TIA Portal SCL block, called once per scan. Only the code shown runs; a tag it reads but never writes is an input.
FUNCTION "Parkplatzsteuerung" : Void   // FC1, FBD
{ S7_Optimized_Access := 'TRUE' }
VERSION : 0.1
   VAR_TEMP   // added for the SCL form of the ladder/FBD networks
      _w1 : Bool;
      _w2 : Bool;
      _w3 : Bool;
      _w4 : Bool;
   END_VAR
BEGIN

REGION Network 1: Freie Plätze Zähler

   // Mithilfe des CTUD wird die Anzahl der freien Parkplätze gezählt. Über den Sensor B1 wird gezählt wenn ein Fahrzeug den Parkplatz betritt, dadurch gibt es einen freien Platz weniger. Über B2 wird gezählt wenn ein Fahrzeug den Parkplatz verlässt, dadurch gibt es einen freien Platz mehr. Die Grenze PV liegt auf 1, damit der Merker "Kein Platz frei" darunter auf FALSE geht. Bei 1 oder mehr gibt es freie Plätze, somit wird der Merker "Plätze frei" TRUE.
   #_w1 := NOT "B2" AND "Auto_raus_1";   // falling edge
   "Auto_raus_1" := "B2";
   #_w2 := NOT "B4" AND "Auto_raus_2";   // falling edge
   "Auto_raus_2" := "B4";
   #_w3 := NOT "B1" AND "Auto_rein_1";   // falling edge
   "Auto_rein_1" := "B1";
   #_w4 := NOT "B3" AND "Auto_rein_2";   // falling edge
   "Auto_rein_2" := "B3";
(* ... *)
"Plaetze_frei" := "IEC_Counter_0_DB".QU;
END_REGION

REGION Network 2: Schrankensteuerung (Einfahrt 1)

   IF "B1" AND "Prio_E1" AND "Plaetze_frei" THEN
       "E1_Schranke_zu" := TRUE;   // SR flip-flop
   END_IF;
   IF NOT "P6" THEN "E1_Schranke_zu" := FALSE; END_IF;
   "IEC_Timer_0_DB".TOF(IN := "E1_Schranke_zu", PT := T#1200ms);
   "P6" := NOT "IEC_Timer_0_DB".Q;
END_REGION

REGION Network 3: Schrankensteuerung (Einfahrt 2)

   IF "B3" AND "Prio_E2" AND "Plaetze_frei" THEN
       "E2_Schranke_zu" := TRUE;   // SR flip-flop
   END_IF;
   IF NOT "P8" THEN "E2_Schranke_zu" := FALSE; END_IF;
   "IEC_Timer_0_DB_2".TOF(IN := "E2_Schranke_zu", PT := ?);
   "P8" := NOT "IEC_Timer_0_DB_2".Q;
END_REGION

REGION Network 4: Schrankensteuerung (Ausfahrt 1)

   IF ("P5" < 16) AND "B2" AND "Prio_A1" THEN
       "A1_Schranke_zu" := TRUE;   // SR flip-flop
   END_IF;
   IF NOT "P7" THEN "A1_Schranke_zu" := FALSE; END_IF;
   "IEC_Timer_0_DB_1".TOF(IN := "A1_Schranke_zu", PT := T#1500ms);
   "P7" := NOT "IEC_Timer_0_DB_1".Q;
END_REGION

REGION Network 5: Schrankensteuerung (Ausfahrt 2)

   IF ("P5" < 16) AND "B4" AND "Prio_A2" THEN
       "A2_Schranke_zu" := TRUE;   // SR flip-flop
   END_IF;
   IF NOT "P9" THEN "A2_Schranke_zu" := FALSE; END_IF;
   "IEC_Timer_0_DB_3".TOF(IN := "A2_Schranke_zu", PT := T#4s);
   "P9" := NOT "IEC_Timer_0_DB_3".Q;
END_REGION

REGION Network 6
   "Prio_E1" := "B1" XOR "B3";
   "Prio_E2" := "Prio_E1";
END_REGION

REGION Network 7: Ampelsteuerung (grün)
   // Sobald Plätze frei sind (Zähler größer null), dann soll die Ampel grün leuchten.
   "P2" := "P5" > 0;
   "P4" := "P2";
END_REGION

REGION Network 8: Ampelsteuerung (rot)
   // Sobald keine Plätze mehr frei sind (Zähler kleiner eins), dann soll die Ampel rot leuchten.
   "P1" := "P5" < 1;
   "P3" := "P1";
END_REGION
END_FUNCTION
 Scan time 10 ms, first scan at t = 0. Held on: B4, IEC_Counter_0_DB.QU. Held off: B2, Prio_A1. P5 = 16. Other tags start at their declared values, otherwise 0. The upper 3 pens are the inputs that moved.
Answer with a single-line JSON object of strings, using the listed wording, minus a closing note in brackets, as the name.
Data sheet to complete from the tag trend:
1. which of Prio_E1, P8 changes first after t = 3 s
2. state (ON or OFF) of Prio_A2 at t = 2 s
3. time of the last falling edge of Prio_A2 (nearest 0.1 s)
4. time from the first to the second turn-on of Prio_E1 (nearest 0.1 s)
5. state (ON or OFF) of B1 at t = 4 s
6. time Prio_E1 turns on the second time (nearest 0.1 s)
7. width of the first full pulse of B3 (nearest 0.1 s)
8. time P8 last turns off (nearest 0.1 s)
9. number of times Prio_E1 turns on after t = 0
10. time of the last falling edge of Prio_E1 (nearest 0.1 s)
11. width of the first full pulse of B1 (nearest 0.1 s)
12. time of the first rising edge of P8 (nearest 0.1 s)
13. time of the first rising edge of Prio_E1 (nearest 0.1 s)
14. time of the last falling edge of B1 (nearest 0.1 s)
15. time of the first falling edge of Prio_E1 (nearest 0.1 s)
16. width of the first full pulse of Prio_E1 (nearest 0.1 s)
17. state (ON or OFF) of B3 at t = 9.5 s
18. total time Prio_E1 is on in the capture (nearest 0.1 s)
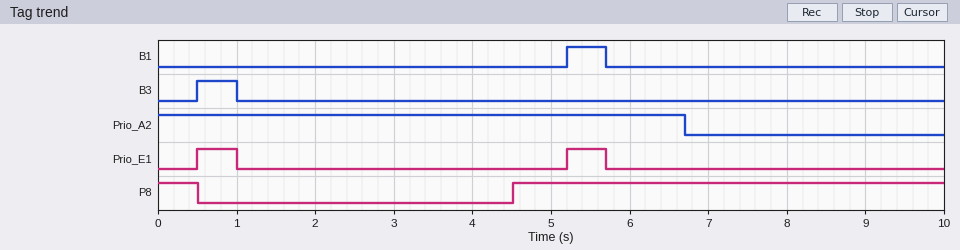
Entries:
{"which of Prio_E1, P8 changes first after t = 3 s": "P8", "state (ON or OFF) of Prio_A2 at t = 2 s": "ON", "time of the last falling edge of Prio_A2": "6.7 s", "time from the first to the second turn-on of Prio_E1": "4.7 s", "state (ON or OFF) of B1 at t = 4 s": "OFF", "time Prio_E1 turns on the second time": "5.2 s", "width of the first full pulse of B3": "0.5 s", "time P8 last turns off": "0.5 s", "number of times Prio_E1 turns on after t = 0": "2", "time of the last falling edge of Prio_E1": "5.7 s", "width of the first full pulse of B1": "0.5 s", "time of the first rising edge of P8": "4.5 s", "time of the first rising edge of Prio_E1": "0.5 s", "time of the last falling edge of B1": "5.7 s", "time of the first falling edge of Prio_E1": "1.0 s", "width of the first full pulse of Prio_E1": "0.5 s", "state (ON or OFF) of B3 at t = 9.5 s": "OFF", "total time Prio_E1 is on in the capture": "1.0 s"}
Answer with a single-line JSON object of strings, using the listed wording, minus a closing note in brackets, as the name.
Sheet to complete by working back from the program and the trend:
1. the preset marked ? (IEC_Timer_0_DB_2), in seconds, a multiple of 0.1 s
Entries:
{"the preset marked ? (IEC_Timer_0_DB_2), in seconds, a multiple of 0.1 s": "4.0 s"}
